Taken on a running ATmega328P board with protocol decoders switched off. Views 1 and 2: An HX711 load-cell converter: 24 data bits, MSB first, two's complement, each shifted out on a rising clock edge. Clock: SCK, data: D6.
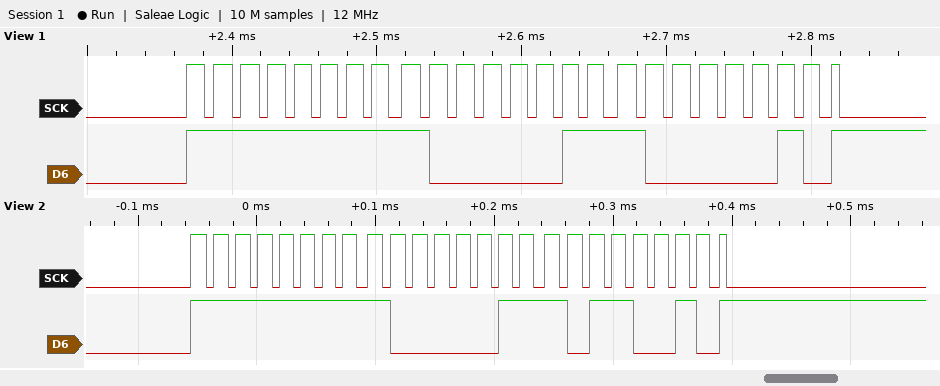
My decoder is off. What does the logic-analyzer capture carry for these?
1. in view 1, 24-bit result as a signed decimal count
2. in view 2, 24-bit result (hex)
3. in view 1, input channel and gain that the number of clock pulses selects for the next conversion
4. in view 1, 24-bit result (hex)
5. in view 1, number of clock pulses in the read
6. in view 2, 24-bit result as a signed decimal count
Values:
-31870
0xFF83B2
channel A, gain 128
0xFF8382
25
-31822
